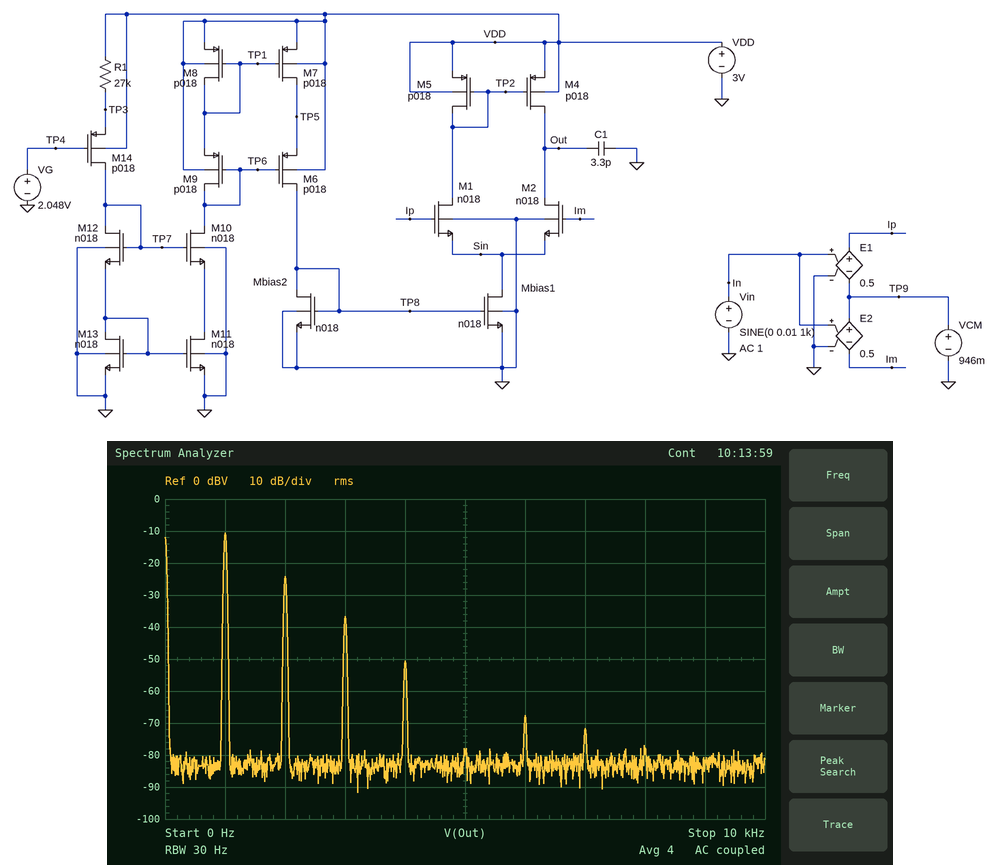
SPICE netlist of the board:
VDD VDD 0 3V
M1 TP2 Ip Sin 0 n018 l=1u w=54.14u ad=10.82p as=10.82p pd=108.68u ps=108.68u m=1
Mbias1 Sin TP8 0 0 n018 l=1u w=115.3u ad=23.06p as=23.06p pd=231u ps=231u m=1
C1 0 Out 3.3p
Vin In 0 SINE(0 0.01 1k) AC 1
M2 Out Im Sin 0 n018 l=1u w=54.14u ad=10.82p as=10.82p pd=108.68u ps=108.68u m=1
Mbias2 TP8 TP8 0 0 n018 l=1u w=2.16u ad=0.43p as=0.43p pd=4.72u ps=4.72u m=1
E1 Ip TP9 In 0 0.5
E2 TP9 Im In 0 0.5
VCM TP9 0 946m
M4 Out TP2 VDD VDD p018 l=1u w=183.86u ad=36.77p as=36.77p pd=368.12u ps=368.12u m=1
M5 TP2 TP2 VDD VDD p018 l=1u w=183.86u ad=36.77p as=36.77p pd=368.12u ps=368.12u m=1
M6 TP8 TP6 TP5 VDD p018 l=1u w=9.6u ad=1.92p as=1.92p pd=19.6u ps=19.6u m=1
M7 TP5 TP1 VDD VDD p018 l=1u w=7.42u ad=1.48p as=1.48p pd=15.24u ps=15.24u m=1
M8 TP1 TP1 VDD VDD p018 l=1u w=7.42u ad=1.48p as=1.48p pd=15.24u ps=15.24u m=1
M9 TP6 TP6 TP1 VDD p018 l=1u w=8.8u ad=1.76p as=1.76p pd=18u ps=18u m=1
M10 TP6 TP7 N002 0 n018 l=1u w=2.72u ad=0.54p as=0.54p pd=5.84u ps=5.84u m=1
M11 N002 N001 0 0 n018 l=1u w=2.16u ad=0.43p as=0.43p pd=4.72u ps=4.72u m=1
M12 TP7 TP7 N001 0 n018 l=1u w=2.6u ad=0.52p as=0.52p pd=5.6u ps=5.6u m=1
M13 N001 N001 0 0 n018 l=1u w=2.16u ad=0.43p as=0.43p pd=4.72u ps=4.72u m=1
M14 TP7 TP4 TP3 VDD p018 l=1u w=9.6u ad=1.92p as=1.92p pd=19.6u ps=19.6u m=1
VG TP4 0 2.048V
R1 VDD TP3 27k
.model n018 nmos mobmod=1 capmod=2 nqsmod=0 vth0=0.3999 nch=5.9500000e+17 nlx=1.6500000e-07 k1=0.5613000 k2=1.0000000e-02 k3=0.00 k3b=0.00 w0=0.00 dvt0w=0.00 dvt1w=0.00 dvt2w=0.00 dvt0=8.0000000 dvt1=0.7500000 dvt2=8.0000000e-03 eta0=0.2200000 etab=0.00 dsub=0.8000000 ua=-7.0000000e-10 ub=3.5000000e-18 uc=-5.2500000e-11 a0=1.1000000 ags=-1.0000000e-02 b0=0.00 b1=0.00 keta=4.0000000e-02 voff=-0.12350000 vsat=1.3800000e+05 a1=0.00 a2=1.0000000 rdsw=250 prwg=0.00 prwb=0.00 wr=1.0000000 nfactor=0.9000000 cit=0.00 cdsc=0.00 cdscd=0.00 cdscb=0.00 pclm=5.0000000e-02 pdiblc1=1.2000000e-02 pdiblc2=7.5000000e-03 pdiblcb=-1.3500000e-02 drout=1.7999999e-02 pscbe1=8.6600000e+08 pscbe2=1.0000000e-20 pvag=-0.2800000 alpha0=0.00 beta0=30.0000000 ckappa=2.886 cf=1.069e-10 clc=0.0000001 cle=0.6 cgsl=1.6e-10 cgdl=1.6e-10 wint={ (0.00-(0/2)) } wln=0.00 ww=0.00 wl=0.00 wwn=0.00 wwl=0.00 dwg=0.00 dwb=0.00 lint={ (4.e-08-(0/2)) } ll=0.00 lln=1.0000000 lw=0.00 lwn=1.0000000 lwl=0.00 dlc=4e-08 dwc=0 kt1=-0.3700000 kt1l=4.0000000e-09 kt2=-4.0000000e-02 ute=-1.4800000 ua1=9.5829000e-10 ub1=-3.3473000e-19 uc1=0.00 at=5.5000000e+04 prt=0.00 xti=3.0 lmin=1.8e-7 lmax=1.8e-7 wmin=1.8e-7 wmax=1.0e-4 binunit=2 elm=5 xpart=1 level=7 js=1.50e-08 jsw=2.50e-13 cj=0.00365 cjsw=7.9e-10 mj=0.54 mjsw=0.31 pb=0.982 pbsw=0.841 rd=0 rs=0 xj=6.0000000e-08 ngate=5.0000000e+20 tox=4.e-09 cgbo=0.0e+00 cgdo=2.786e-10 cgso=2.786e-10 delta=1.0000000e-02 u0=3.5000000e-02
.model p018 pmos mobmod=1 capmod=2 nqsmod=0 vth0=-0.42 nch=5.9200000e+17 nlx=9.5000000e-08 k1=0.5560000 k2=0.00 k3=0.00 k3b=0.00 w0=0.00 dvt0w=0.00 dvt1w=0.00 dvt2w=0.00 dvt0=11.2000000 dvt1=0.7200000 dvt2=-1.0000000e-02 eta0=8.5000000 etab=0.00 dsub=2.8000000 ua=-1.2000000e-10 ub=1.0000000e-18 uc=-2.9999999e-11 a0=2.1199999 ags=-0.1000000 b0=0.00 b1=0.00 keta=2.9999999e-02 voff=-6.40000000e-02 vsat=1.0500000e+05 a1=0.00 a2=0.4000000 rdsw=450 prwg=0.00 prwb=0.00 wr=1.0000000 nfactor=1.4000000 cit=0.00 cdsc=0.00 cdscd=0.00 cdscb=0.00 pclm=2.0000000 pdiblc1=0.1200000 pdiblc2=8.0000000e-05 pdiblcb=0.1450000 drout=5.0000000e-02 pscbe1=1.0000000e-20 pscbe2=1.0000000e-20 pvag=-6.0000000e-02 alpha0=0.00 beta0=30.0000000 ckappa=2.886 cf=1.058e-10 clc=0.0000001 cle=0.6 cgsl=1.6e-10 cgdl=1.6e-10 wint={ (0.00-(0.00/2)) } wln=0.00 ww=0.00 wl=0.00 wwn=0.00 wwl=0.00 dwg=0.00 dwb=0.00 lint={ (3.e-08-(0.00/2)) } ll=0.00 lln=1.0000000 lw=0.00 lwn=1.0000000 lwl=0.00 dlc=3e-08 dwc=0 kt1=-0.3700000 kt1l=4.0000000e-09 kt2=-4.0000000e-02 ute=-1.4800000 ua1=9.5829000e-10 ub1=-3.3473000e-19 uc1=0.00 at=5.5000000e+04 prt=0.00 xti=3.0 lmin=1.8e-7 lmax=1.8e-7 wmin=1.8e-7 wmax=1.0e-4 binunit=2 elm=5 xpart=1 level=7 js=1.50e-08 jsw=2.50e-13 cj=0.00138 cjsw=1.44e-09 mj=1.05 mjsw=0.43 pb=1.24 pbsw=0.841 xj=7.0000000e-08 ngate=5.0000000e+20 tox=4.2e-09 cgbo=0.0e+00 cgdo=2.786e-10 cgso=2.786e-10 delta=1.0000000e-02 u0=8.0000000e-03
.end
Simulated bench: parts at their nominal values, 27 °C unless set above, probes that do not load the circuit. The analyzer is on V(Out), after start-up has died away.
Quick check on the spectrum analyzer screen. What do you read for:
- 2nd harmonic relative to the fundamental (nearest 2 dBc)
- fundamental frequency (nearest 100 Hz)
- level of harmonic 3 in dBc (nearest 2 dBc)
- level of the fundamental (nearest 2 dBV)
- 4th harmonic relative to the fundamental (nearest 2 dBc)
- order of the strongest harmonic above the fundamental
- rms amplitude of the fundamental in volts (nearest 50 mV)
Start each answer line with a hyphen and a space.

- -14 dBc
- 1.0 kHz
- -26 dBc
- -10 dBV
- -40 dBc
- 2
- 300 mV
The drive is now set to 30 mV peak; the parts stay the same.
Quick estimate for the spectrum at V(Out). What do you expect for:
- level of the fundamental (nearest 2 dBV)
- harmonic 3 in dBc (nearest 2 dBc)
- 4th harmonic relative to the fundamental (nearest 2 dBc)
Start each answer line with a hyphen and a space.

- -2 dBV
- -20 dBc
- -20 dBc
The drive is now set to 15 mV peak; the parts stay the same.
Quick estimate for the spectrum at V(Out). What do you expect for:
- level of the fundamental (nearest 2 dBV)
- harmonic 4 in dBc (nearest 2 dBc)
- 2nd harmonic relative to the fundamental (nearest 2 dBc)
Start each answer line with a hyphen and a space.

- -6 dBV
- -38 dBc
- -12 dBc
